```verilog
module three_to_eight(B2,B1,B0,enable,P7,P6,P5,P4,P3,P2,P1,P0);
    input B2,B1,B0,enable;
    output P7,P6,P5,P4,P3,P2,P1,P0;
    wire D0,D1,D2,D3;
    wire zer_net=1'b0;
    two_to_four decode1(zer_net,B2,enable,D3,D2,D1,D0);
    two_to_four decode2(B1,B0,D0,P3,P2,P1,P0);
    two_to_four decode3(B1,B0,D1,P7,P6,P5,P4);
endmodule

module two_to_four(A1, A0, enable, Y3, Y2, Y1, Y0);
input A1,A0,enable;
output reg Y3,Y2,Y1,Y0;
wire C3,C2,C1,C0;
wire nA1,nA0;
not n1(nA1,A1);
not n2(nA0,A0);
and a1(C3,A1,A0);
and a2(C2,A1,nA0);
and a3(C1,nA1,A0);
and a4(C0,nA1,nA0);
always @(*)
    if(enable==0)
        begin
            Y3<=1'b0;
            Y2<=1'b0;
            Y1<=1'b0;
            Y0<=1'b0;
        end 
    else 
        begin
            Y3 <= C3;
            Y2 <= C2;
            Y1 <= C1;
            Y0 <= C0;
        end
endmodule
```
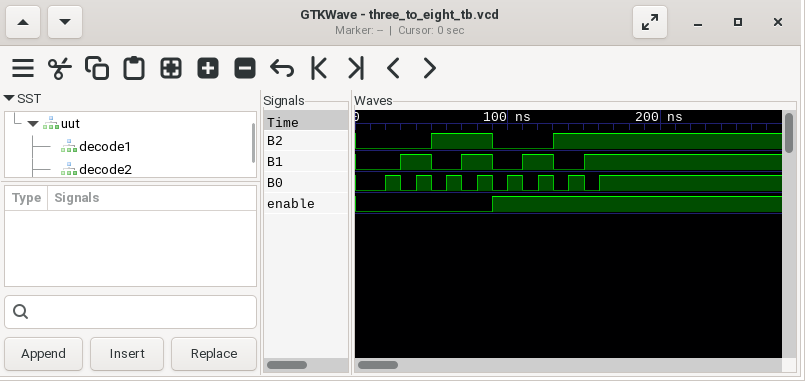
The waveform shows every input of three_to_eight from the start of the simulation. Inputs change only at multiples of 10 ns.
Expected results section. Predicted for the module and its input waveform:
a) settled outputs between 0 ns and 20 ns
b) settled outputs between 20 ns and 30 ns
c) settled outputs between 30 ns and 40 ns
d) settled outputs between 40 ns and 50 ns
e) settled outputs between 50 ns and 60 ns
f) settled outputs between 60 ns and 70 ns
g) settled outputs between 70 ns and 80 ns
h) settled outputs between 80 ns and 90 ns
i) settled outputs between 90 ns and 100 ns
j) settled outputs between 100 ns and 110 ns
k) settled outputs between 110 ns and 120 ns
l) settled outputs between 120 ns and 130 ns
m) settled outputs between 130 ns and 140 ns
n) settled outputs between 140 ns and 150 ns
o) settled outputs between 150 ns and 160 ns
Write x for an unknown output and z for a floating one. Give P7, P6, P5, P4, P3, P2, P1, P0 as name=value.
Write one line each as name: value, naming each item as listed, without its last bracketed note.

settled outputs between 0 ns and 20 ns: P7=0, P6=0, P5=0, P4=0, P3=0, P2=0, P1=0, P0=0
settled outputs between 20 ns and 30 ns: P7=0, P6=0, P5=0, P4=0, P3=0, P2=0, P1=0, P0=0
settled outputs between 30 ns and 40 ns: P7=0, P6=0, P5=0, P4=0, P3=0, P2=0, P1=0, P0=0
settled outputs between 40 ns and 50 ns: P7=0, P6=0, P5=0, P4=0, P3=0, P2=0, P1=0, P0=0
settled outputs between 50 ns and 60 ns: P7=0, P6=0, P5=0, P4=0, P3=0, P2=0, P1=0, P0=0
settled outputs between 60 ns and 70 ns: P7=0, P6=0, P5=0, P4=0, P3=0, P2=0, P1=0, P0=0
settled outputs between 70 ns and 80 ns: P7=0, P6=0, P5=0, P4=0, P3=0, P2=0, P1=0, P0=0
settled outputs between 80 ns and 90 ns: P7=0, P6=0, P5=0, P4=0, P3=0, P2=0, P1=0, P0=0
settled outputs between 90 ns and 100 ns: P7=0, P6=0, P5=0, P4=0, P3=0, P2=0, P1=0, P0=1
settled outputs between 100 ns and 110 ns: P7=0, P6=0, P5=0, P4=0, P3=0, P2=0, P1=1, P0=0
settled outputs between 110 ns and 120 ns: P7=0, P6=0, P5=0, P4=0, P3=0, P2=1, P1=0, P0=0
settled outputs between 120 ns and 130 ns: P7=0, P6=0, P5=0, P4=0, P3=1, P2=0, P1=0, P0=0
settled outputs between 130 ns and 140 ns: P7=0, P6=0, P5=0, P4=1, P3=0, P2=0, P1=0, P0=0
settled outputs between 140 ns and 150 ns: P7=0, P6=0, P5=1, P4=0, P3=0, P2=0, P1=0, P0=0
settled outputs between 150 ns and 160 ns: P7=0, P6=1, P5=0, P4=0, P3=0, P2=0, P1=0, P0=0
